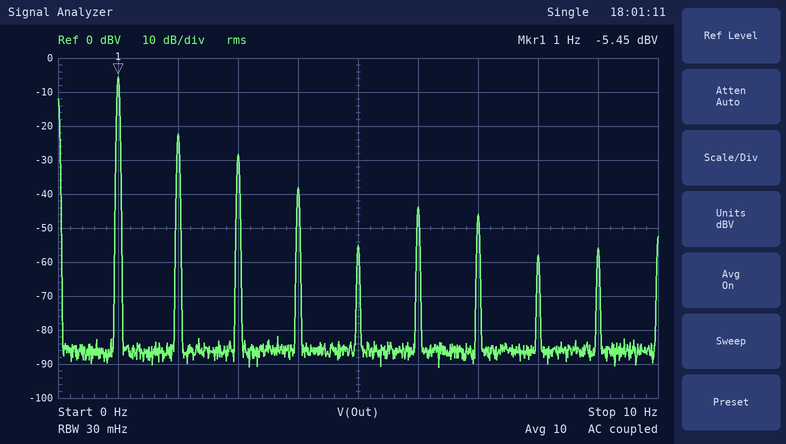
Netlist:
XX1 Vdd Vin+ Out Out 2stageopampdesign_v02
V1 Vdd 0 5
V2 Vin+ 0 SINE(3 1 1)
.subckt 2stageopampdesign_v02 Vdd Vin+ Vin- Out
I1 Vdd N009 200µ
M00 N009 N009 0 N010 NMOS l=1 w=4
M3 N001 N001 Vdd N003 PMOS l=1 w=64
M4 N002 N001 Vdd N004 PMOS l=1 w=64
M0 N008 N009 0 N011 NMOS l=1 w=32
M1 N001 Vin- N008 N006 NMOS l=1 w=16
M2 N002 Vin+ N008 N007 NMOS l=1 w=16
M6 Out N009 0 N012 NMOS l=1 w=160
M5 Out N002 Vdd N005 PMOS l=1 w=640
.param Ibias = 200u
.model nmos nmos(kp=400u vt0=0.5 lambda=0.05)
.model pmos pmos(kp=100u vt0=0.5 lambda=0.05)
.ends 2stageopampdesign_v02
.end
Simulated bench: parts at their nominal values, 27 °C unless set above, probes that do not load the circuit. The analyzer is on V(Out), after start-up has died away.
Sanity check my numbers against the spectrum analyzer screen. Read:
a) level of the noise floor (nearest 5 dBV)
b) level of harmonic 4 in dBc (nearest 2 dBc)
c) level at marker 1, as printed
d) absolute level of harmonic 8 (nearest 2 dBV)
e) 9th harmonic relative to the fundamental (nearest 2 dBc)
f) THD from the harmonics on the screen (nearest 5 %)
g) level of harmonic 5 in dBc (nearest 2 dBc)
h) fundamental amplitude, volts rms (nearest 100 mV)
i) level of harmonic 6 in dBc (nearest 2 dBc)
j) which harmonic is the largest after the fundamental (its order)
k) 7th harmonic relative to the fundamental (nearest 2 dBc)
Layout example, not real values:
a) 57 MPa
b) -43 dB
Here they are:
a) -85 dBV
b) -32 dBc
c) -5.45 dBV
d) -58 dBV
e) -50 dBc
f) 15 %
g) -50 dBc
h) 500 mV
i) -38 dBc
j) 2
k) -40 dBc
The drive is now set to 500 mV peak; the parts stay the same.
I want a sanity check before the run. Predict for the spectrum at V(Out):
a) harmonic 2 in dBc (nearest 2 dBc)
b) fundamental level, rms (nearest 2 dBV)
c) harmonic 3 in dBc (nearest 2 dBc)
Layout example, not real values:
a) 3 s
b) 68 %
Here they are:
a) -36 dBc
b) -10 dBV
c) -48 dBc
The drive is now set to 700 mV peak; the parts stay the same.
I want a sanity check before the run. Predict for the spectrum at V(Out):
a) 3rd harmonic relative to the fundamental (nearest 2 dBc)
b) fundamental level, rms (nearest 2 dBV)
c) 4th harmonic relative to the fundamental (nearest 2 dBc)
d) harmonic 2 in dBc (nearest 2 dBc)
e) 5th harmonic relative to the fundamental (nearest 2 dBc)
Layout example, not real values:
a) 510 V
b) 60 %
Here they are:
a) -32 dBc
b) -8 dBV
c) -36 dBc
d) -26 dBc
e) -40 dBc
